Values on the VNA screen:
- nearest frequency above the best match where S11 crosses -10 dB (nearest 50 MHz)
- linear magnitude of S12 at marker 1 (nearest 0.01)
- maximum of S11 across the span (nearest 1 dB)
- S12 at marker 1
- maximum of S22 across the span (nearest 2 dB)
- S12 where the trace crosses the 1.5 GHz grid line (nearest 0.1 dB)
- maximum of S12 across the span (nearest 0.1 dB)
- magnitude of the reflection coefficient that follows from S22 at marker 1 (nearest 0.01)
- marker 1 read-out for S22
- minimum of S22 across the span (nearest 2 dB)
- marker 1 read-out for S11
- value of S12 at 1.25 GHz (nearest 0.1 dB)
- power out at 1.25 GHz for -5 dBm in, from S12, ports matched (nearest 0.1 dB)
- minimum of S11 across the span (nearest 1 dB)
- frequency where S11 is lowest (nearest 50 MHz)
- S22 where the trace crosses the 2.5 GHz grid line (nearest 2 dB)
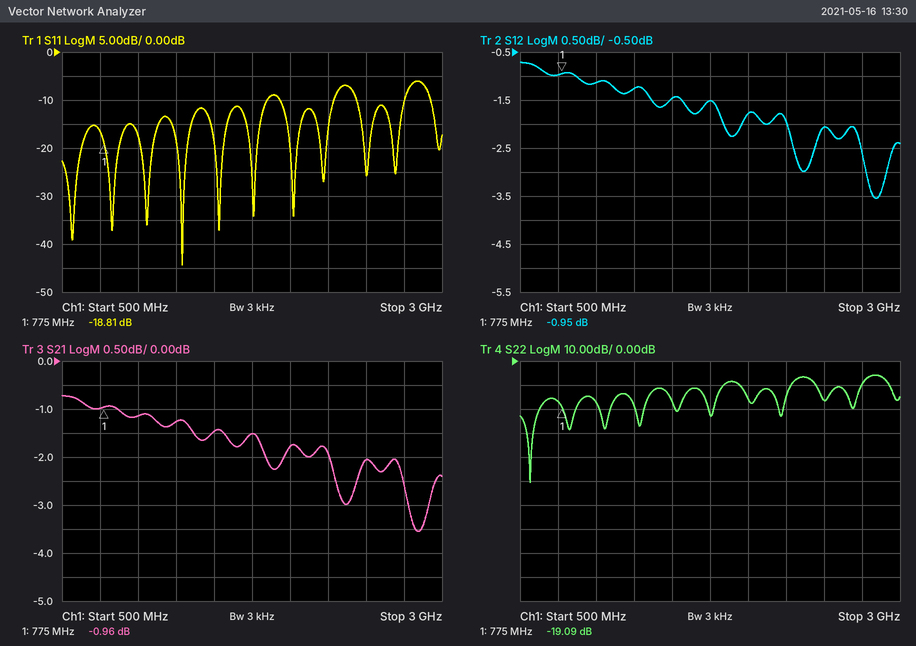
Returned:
1.85 GHz
0.90
-6 dB
-0.95 dB
-6 dB
-1.5 dB
-0.7 dB
0.11
-19.09 dB
-50 dB
-18.81 dB
-1.3 dB
-6.3 dBm
-44 dB
1.30 GHz
-16 dB
